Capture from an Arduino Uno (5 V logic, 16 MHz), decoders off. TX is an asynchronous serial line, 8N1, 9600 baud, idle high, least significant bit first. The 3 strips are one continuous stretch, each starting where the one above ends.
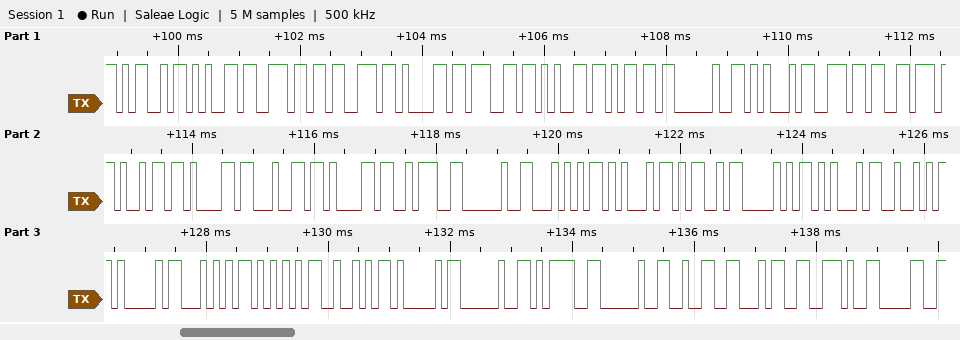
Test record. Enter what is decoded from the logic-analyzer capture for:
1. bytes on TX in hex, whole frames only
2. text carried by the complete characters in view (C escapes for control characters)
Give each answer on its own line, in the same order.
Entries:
4D 65 6E 73 61 67 65 6D 20 45 6E 76 69 61 64 61 3A 20 54 45 4D 50 45 52 41 54 55 52 41 20 3D 20 32 34 2E 30
"Mensagem Enviada: TEMPERATURA = 24.0"
